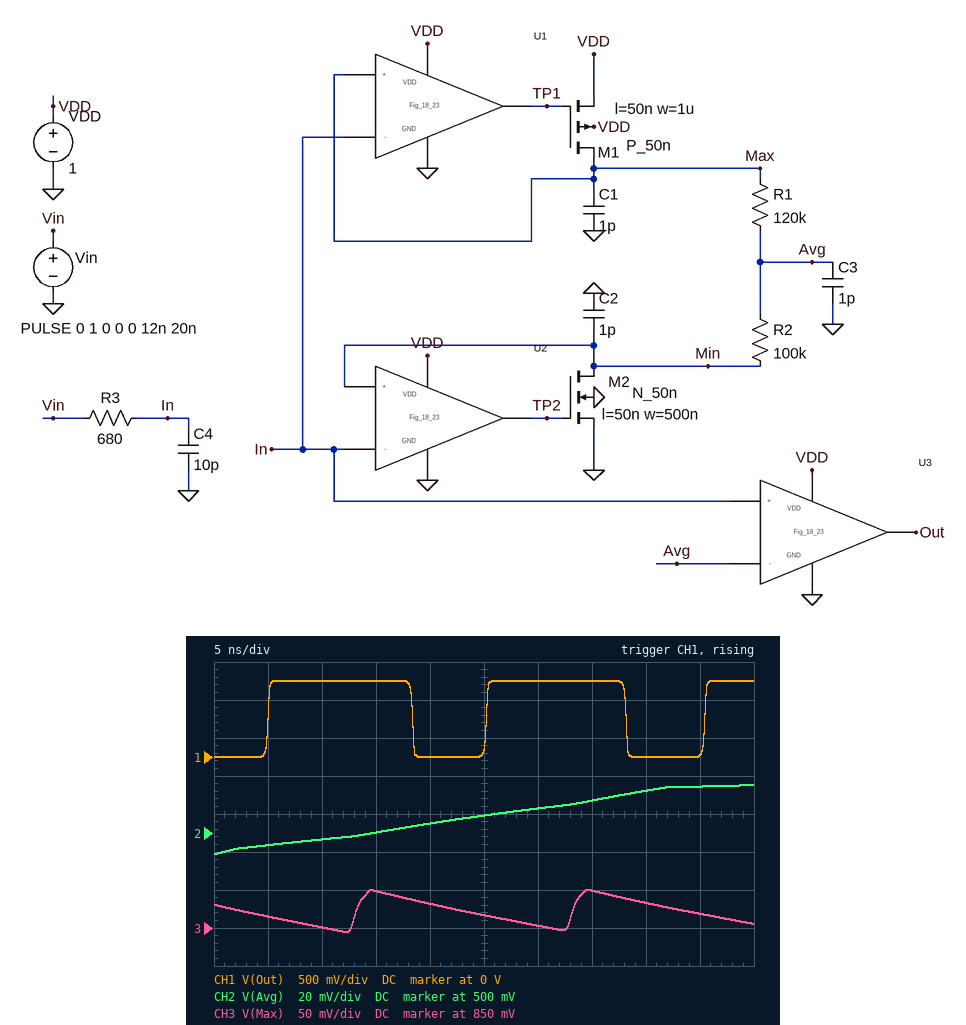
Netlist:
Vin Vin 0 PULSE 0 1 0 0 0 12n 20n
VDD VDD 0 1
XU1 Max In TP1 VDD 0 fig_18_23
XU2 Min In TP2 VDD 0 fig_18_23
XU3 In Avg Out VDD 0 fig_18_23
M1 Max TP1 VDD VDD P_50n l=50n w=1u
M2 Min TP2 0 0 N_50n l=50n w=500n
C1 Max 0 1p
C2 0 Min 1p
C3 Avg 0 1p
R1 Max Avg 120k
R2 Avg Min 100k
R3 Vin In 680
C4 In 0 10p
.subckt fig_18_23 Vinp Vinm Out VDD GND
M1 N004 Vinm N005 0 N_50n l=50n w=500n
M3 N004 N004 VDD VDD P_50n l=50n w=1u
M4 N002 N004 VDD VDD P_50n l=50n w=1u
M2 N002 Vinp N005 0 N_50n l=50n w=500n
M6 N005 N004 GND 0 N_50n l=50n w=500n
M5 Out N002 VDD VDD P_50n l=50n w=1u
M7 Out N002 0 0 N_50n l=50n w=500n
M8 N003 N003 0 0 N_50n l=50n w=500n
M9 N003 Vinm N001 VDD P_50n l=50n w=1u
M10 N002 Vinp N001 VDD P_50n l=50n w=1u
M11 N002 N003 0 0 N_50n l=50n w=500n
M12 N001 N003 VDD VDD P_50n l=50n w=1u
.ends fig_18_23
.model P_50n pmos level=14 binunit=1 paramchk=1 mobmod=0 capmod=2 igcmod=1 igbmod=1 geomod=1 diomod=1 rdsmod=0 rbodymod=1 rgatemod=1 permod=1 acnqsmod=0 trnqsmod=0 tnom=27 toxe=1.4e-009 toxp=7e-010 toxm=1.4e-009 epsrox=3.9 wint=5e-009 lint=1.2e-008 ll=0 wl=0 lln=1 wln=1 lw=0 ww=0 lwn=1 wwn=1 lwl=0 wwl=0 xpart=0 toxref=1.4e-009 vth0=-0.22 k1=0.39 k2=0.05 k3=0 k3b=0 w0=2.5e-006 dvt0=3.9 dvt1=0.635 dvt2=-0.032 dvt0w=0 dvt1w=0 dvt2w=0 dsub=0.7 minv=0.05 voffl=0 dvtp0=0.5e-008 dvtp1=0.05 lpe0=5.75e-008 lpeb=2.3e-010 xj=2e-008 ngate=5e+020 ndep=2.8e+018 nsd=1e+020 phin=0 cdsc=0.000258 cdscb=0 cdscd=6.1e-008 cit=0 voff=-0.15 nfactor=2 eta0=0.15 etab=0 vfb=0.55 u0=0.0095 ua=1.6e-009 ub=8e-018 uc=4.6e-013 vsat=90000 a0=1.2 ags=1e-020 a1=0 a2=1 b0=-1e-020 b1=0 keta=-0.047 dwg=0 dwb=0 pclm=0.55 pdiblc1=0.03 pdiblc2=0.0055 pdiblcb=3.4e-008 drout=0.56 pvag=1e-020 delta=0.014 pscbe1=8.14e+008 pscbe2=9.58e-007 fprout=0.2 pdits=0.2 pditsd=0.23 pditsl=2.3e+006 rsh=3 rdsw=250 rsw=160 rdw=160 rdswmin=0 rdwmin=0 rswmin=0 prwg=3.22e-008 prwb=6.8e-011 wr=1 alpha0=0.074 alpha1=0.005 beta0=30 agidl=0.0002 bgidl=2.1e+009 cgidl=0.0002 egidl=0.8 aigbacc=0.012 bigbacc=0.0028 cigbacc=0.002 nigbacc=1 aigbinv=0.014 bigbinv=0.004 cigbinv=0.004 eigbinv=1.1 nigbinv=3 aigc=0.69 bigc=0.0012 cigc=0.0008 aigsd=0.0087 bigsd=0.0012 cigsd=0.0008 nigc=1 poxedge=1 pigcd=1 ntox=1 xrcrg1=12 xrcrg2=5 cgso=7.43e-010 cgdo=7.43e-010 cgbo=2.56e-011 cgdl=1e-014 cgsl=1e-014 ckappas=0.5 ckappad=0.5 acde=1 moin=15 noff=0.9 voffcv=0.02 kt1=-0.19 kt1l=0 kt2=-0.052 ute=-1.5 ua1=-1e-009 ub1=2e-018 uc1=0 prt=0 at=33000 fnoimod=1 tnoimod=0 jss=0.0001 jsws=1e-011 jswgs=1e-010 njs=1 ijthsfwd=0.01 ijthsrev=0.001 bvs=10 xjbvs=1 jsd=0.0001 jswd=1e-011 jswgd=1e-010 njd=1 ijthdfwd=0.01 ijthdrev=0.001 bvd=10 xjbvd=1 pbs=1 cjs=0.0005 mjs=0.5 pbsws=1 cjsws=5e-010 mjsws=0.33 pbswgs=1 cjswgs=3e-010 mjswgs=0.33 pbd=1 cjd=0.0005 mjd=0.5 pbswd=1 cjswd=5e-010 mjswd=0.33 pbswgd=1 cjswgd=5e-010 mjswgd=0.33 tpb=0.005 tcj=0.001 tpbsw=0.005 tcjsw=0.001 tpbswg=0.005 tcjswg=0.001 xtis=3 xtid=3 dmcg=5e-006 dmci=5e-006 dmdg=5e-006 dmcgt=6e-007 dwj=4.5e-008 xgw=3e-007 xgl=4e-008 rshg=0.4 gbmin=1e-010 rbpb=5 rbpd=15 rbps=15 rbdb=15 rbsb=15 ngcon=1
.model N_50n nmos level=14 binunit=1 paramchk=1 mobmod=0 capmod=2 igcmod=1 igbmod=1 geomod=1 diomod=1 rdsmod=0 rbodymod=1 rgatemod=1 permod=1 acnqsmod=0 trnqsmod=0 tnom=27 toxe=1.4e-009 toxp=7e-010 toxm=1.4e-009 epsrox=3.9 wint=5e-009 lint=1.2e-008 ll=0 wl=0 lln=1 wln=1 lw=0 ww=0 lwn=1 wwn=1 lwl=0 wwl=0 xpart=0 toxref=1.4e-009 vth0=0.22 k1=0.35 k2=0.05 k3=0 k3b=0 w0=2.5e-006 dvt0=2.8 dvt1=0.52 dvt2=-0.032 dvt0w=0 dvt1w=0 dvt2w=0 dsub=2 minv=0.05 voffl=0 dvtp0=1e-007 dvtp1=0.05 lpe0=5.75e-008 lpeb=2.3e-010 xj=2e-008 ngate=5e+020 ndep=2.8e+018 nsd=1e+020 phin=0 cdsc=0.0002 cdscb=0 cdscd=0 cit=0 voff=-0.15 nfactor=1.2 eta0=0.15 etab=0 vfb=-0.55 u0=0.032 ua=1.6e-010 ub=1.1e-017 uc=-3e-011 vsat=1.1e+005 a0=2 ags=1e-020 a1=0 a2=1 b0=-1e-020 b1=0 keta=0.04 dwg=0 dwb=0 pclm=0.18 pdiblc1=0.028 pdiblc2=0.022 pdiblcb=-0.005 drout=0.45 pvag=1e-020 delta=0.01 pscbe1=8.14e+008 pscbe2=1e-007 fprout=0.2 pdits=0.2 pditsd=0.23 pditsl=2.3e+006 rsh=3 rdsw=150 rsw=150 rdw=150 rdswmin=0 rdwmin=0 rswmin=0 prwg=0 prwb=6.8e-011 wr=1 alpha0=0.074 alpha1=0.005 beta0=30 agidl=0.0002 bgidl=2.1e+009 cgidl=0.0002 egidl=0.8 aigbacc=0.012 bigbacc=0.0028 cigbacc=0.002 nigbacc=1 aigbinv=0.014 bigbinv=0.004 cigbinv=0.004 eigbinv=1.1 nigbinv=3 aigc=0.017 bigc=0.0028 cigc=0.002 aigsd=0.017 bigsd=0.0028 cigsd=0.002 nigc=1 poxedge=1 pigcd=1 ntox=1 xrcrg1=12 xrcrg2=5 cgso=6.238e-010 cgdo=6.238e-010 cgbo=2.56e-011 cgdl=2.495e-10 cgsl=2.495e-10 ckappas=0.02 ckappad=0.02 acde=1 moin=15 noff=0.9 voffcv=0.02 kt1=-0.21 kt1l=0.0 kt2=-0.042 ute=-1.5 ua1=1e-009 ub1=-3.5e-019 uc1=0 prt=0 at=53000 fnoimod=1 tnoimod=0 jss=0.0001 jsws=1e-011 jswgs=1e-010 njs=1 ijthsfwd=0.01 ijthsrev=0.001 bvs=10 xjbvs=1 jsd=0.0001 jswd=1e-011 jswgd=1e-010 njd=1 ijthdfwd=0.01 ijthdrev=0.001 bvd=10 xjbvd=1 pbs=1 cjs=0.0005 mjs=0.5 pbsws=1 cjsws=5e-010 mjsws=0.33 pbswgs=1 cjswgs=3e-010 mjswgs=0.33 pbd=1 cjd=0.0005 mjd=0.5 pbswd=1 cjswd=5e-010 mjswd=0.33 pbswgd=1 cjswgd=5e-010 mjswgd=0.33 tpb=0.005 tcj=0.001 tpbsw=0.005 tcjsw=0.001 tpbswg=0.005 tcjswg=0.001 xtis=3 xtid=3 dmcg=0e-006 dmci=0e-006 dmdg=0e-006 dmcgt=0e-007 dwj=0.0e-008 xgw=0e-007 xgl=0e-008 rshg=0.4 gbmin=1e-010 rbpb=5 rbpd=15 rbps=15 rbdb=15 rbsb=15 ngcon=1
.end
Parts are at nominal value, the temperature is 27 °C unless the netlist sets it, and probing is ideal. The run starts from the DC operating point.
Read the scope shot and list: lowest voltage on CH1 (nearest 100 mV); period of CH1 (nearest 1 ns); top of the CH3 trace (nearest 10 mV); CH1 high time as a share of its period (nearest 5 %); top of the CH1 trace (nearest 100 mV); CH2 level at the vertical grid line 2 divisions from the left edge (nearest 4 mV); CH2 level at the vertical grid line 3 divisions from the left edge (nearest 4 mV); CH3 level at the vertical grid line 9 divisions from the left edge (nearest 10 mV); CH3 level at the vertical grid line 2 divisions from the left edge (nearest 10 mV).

0 V
20 ns
900 mV
65 %
1.0 V
496 mV
500 mV
870 mV
850 mV
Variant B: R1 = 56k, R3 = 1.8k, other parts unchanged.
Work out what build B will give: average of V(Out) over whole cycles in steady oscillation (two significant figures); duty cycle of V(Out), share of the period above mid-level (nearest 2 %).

550 mV
54 %
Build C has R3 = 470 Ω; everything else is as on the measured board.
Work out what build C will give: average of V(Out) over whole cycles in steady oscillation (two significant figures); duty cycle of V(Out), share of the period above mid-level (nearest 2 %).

630 mV
62 %
